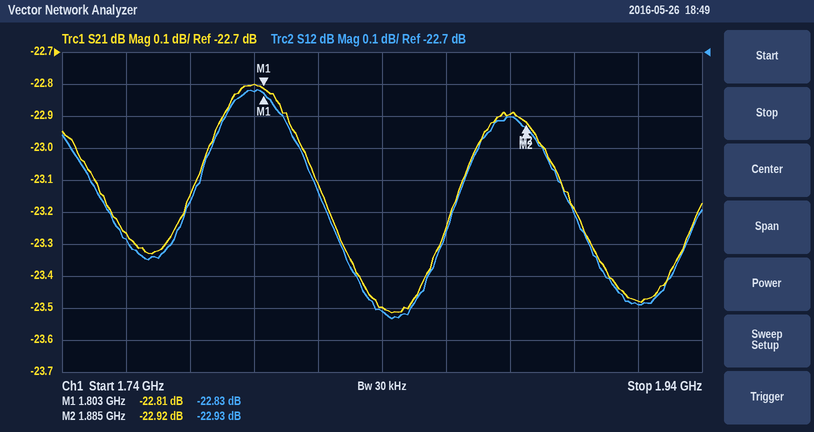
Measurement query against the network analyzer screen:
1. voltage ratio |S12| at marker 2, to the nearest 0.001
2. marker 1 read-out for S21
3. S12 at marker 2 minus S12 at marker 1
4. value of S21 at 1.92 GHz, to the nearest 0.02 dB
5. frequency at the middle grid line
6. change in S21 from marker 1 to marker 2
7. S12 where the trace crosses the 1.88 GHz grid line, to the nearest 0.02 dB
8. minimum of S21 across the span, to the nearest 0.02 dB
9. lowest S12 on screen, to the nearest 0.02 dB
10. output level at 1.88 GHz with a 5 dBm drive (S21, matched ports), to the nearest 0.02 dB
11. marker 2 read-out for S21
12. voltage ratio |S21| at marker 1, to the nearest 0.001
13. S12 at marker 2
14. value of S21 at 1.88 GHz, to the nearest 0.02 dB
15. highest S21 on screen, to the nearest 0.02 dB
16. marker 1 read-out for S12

0.071
-22.81 dB
-0.10 dB
-23.48 dB
1.84 GHz
-0.11 dB
-22.90 dB
-23.52 dB
-23.54 dB
-17.90 dBm
-22.92 dB
0.072
-22.93 dB
-22.90 dB
-22.80 dB
-22.83 dB
